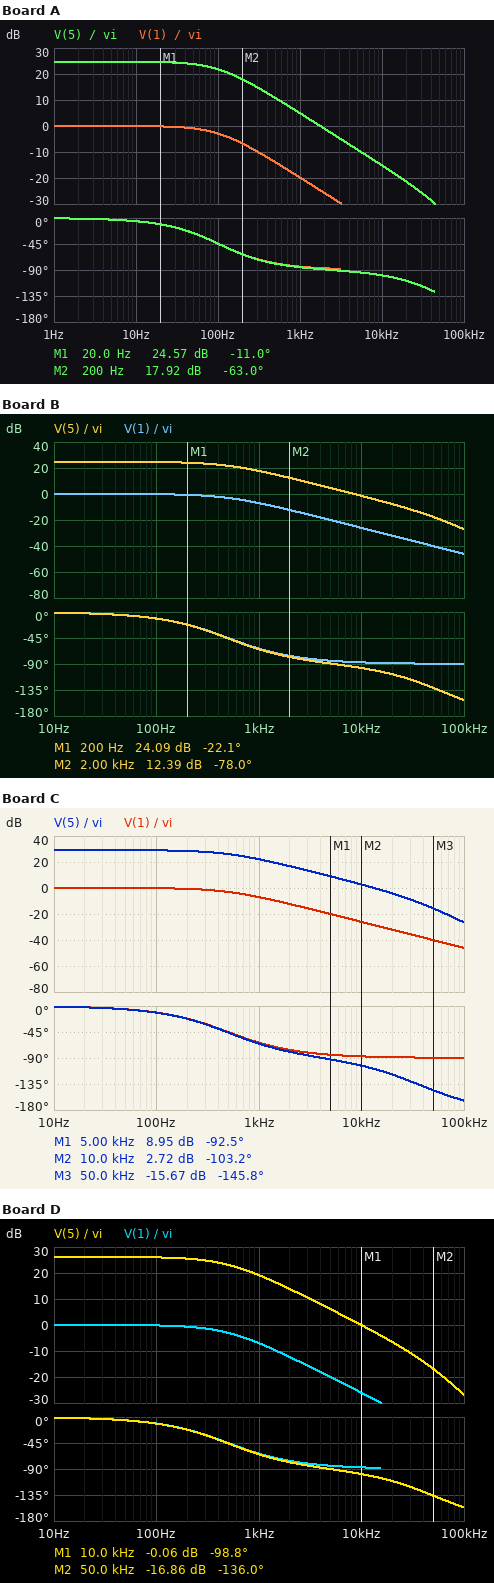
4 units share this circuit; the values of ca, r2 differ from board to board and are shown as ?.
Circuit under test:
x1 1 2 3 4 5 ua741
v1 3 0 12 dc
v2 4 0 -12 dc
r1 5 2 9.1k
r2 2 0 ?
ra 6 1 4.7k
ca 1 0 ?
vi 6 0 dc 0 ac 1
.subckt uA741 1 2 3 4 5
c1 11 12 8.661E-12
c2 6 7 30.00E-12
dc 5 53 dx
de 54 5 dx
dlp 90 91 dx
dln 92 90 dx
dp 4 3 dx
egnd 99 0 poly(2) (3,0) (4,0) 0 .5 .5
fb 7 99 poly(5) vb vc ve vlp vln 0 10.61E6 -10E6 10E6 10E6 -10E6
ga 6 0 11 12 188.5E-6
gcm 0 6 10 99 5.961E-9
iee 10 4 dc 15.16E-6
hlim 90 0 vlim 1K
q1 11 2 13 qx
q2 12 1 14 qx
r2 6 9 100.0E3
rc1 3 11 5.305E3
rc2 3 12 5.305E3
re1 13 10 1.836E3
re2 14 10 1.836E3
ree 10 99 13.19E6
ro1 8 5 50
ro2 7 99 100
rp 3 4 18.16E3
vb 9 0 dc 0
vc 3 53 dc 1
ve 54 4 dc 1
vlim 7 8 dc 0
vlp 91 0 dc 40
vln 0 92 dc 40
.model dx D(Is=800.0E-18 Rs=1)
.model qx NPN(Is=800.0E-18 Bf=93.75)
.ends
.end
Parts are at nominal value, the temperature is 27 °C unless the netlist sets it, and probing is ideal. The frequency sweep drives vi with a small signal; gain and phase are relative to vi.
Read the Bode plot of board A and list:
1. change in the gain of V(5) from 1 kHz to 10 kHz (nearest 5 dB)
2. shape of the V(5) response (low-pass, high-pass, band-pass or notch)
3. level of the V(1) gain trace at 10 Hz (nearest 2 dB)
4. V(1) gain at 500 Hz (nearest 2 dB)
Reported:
-20 dB
low-pass
0 dB
-14 dB
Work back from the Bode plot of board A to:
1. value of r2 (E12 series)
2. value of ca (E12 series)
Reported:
560 Ω
330 nF
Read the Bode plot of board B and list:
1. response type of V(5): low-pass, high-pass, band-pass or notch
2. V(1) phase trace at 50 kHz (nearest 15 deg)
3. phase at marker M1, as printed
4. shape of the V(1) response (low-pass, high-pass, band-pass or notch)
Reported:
low-pass
-90 deg
-22.1 deg
low-pass
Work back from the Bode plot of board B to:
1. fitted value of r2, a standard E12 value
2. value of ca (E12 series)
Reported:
560 Ω
68 nF
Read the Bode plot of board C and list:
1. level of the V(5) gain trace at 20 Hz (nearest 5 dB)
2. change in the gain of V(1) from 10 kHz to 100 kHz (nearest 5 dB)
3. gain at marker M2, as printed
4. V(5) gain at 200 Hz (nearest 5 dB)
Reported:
30 dB
-20 dB
2.72 dB
30 dB
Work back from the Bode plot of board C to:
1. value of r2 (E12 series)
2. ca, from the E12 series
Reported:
330 Ω
68 nF
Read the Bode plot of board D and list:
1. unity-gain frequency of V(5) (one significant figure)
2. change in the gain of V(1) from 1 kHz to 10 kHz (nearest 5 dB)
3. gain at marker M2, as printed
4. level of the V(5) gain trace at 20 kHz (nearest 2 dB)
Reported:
10 kHz
-20 dB
-16.86 dB
-6 dB
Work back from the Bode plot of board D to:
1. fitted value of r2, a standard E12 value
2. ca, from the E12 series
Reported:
470 Ω
68 nF
